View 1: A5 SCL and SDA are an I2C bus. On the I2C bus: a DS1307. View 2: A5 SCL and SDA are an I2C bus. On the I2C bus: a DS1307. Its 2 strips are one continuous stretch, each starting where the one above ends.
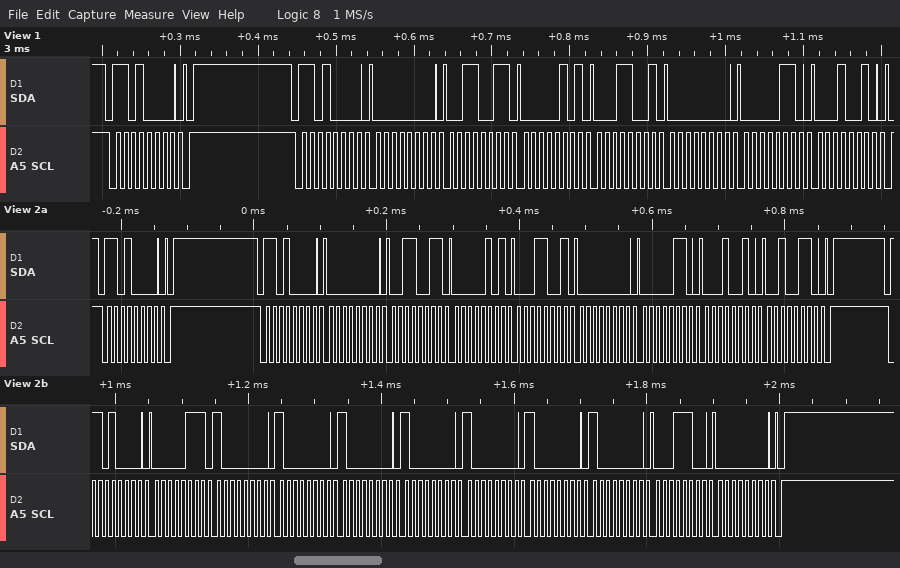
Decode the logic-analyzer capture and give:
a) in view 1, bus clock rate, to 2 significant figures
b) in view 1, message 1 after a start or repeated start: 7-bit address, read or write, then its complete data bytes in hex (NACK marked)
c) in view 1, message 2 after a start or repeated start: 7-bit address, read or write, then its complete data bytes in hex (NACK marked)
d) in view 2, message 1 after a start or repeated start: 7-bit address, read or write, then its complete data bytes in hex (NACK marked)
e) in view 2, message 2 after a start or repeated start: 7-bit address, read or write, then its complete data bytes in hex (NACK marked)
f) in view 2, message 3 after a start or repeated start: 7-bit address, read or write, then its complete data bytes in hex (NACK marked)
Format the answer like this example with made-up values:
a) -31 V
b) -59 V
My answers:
a) 100 kHz
b) 0x68 write
c) 0x68 write: 00 33 05 19 00 06 12
d) 0x68 write
e) 0x68 write: 00 33 05 19 00 06 12 26
f) 0x68 write: 07 80 80 80 80 80 80 80 1C 00
